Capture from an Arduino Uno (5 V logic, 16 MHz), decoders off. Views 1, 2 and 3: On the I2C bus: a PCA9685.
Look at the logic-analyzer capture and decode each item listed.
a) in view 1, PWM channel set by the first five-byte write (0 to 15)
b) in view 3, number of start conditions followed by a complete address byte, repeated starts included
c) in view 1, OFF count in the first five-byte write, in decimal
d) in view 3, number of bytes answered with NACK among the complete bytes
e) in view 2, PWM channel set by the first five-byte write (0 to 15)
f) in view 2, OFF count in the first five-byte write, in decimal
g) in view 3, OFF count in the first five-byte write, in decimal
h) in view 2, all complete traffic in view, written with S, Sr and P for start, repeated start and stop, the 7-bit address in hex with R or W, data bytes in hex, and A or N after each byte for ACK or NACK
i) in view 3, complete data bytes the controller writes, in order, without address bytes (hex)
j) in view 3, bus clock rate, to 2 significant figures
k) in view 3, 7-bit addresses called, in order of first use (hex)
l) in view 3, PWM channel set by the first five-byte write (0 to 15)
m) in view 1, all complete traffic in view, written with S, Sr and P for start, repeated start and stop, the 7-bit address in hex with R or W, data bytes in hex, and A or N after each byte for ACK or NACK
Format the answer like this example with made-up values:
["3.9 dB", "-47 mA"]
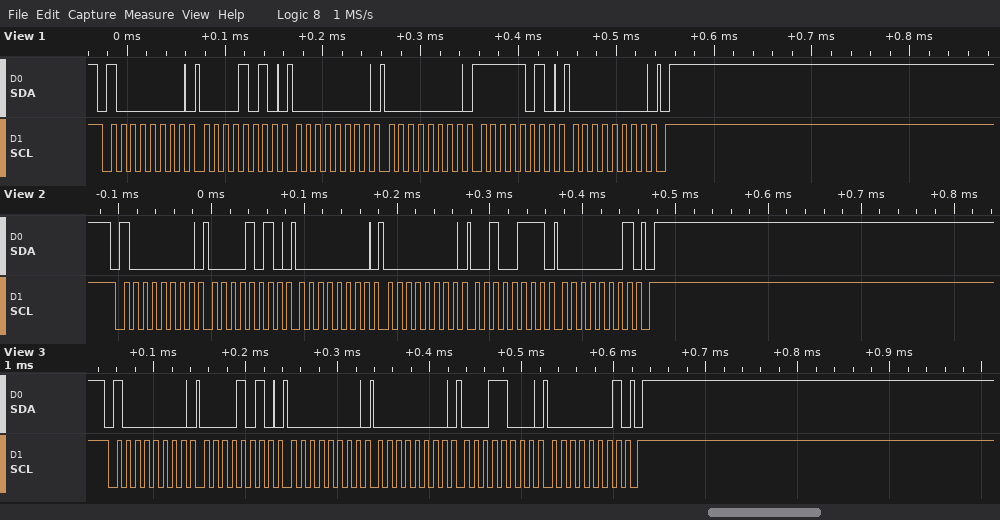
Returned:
["1", "1", "250", "0", "1", "295", "280", "S 40W A 0A A 00 A 00 A 27 A 01 A P", "0A 00 00 18 01", "100 kHz", "0x40", "1", "S 40W A 0A A 00 A 00 A FA A 00 A P"]
